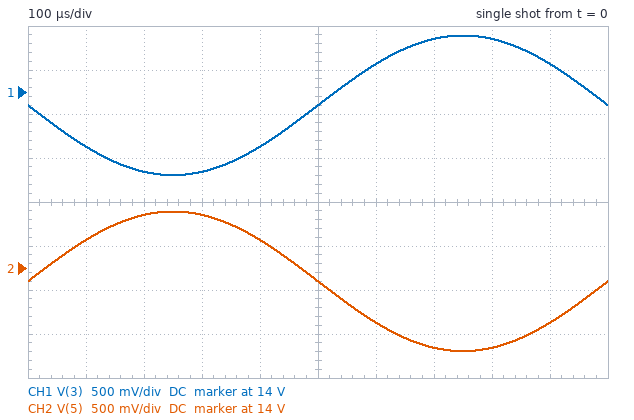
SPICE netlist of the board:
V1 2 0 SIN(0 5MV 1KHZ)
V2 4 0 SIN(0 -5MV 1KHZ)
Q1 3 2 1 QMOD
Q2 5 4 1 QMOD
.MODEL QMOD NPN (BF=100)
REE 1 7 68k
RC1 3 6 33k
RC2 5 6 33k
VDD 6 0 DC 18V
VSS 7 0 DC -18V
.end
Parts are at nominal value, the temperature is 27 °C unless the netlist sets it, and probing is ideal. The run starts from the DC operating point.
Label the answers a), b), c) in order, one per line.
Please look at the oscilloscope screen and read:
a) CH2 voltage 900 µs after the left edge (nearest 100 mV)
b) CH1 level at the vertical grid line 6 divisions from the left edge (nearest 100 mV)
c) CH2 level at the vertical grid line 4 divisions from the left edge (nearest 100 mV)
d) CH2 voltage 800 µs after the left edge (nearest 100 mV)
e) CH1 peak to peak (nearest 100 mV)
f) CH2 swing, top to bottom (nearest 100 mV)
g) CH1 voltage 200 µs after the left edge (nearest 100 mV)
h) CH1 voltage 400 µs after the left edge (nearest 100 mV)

a) 13.4 V
b) 14.3 V
c) 14.3 V
d) 13.1 V
e) 1.6 V
f) 1.6 V
g) 13.1 V
h) 13.4 V
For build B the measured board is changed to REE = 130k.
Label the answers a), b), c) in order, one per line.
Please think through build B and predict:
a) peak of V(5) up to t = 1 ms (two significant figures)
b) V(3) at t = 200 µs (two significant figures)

a) 16 V
b) 15 V
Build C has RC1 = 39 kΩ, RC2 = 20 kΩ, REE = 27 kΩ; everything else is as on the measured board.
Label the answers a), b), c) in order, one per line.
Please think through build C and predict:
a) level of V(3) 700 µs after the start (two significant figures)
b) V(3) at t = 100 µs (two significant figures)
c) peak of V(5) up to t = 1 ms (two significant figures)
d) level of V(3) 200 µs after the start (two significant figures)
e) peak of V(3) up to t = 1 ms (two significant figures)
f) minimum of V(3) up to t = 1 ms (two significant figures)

a) 7.9 V
b) 4.3 V
c) 13 V
d) 3.4 V
e) 8.0 V
f) 3.3 V
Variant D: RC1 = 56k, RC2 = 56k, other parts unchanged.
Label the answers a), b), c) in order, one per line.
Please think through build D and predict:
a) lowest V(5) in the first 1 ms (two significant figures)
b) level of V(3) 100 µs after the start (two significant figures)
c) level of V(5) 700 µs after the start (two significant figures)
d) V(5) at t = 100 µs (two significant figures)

a) 9.6 V
b) 10 V
c) 9.7 V
d) 12 V
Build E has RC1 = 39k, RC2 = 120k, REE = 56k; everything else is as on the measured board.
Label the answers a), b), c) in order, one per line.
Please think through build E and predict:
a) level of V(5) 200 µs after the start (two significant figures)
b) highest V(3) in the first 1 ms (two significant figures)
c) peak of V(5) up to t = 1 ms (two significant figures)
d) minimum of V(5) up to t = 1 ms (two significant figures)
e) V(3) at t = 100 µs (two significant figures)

a) 3.0 V
b) 13 V
c) 3.2 V
d) -670 mV
e) 11 V
